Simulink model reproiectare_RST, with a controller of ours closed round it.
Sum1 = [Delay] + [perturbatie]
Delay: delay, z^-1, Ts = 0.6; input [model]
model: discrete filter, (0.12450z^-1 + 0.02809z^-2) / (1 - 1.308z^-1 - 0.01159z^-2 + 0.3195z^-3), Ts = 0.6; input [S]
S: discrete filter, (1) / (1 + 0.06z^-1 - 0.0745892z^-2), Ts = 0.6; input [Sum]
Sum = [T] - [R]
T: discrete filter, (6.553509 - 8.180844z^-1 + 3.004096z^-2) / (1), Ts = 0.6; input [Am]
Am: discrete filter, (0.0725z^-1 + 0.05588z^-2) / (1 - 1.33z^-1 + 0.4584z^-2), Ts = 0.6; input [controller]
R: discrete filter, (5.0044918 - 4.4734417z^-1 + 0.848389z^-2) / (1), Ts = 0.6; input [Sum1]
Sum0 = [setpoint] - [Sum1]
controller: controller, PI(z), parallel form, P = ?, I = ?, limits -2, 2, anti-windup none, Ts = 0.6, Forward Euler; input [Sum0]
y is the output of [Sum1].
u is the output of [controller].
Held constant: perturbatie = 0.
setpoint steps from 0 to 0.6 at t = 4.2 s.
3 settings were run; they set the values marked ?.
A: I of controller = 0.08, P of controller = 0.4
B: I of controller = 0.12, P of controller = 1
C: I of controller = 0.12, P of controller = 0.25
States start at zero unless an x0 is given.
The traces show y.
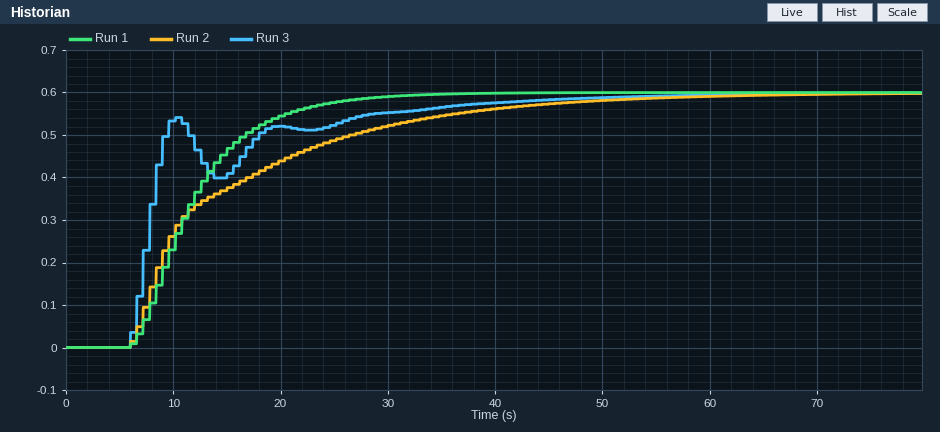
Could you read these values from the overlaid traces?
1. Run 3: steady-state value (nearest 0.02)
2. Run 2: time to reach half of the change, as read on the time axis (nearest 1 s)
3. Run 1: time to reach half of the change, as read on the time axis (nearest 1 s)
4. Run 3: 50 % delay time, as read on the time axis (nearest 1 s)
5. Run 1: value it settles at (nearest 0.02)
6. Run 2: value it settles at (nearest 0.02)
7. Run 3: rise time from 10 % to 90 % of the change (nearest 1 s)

0.60
11 s
11 s
8 s
0.60
0.60
4 s
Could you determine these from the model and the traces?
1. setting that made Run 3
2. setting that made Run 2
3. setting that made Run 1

B
A
C
